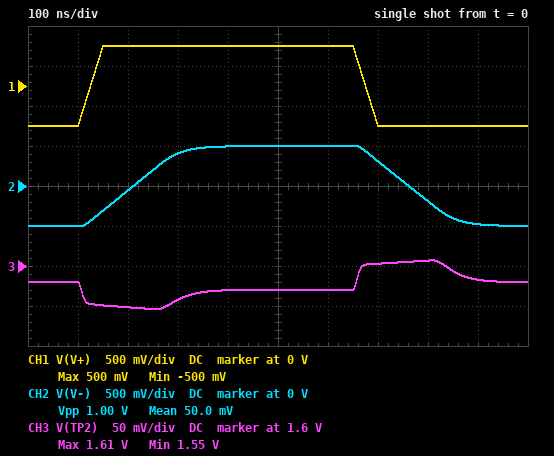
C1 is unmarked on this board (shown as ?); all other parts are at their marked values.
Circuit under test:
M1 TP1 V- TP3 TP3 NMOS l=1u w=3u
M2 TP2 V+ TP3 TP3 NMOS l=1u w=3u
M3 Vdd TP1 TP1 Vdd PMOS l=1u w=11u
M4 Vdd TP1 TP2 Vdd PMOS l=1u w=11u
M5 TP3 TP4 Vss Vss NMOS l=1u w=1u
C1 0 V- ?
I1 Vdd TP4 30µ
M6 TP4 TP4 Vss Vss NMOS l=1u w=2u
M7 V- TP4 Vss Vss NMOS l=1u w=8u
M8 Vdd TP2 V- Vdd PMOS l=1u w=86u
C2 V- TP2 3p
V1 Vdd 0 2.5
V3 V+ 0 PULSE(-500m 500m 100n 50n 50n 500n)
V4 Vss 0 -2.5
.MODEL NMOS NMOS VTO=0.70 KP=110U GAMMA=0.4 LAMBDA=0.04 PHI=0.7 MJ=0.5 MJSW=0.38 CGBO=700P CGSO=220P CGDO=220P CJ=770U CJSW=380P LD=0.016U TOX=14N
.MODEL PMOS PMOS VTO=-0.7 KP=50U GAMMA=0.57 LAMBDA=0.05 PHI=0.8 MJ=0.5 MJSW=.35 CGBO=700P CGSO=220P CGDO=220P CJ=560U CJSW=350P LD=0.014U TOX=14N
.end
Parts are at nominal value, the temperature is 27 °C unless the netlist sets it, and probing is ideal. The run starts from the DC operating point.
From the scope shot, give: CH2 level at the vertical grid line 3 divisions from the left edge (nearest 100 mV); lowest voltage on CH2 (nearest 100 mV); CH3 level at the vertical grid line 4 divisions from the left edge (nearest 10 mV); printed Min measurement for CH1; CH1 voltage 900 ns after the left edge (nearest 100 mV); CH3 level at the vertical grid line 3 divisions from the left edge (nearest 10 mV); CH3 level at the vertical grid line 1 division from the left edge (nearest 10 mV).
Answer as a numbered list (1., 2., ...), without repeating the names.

1. 400 mV
2. -500 mV
3. 1.57 V
4. -500 mV
5. -500 mV
6. 1.56 V
7. 1.58 V
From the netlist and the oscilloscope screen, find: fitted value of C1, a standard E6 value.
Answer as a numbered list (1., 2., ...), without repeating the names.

1. 3.3 pF
